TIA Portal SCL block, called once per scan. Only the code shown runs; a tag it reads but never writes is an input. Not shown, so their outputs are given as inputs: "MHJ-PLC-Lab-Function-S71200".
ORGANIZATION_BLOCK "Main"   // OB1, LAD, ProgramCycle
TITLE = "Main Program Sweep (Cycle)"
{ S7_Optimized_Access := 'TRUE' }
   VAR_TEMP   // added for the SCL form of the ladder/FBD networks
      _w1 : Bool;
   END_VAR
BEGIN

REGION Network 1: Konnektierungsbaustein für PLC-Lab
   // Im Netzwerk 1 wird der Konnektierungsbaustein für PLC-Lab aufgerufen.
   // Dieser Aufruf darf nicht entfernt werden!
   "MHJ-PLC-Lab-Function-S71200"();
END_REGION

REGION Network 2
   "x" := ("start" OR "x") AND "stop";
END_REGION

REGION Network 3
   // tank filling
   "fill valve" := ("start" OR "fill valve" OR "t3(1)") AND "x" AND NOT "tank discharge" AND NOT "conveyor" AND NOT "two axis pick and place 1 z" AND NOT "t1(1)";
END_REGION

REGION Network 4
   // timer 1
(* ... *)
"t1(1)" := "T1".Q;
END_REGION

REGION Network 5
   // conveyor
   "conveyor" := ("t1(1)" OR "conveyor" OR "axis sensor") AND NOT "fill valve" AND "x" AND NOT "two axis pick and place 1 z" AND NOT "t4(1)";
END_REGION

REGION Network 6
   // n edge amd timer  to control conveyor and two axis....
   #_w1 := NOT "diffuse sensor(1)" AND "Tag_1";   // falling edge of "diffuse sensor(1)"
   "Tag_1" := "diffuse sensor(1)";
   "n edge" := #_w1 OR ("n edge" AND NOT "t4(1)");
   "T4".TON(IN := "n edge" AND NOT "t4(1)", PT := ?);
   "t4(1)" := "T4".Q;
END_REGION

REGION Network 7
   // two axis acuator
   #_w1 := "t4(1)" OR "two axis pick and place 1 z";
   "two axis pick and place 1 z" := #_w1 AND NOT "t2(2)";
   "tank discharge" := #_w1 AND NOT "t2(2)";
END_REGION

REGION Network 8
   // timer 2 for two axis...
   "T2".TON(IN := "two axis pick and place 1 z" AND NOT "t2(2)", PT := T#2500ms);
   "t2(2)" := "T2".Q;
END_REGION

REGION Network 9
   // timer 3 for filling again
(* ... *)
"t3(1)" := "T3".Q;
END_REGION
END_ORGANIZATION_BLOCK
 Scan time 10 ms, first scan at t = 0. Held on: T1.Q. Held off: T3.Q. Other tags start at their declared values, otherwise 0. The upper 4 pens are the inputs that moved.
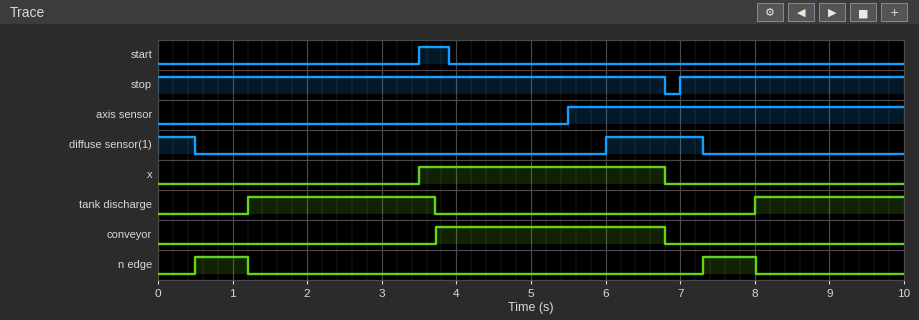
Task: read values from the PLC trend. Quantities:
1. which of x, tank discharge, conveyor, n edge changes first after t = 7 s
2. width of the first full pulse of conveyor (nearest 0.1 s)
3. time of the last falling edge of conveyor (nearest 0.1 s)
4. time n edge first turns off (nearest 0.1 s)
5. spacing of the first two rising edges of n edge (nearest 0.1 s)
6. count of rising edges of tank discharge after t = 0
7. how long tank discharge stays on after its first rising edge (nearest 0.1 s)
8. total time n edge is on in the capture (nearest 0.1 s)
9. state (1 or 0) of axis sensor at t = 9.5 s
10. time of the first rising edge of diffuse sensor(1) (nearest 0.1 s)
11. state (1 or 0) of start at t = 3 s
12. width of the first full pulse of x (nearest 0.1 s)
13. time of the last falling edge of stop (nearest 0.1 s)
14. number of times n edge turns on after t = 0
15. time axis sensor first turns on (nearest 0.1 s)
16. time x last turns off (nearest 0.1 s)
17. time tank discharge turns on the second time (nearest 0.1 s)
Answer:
n edge
3.1 s
6.8 s
1.2 s
6.8 s
2
2.5 s
1.4 s
1
6.0 s
0
3.3 s
6.8 s
2
5.5 s
6.8 s
8.0 s
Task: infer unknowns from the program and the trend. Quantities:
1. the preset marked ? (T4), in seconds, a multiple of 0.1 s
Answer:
0.7 s
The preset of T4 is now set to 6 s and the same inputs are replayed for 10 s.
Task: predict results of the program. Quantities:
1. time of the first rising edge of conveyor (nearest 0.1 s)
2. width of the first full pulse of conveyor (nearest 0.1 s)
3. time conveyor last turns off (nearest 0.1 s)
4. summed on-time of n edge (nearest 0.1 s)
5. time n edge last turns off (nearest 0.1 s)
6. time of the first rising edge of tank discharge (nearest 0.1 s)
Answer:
3.5 s
3.0 s
6.5 s
8.7 s
6.5 s
6.5 s
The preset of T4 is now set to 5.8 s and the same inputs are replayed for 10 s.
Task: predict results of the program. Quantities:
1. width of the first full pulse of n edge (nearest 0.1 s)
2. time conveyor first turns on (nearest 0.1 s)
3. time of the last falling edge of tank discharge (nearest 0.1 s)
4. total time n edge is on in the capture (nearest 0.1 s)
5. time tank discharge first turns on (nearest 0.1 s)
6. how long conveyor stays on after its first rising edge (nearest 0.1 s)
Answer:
5.8 s
3.5 s
8.8 s
8.5 s
6.3 s
2.8 s
